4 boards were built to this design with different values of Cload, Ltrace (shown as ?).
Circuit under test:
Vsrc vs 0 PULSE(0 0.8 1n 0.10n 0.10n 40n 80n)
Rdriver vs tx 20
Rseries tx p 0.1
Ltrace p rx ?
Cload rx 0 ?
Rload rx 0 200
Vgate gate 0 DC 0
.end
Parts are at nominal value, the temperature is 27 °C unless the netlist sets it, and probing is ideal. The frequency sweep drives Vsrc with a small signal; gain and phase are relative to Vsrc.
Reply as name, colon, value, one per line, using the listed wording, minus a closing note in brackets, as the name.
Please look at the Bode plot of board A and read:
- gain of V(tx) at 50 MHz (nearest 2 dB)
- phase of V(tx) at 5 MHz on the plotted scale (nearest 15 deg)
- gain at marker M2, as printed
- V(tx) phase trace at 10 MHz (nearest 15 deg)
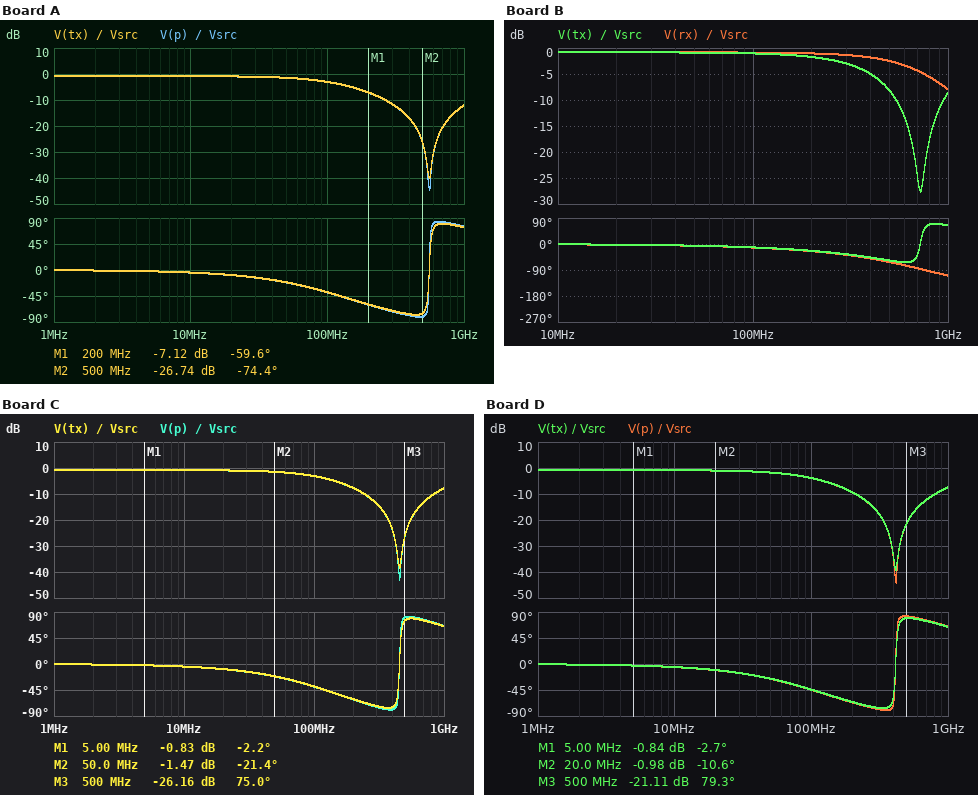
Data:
gain of V(tx) at 50 MHz: -2 dB
phase of V(tx) at 5 MHz on the plotted scale: 0 deg
gain at marker M2, as printed: -26.74 dB
V(tx) phase trace at 10 MHz: 0 deg
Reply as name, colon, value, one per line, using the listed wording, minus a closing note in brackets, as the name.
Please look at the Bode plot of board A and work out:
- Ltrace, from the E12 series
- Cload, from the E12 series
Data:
Ltrace, from the E12 series: 1.2 nH
Cload, from the E12 series: 68 pF
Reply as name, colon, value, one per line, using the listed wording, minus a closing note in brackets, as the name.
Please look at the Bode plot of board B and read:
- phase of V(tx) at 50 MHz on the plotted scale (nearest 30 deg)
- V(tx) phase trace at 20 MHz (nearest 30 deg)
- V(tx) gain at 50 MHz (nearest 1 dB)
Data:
phase of V(tx) at 50 MHz on the plotted scale: 0 deg
V(tx) phase trace at 20 MHz: 0 deg
V(tx) gain at 50 MHz: -1 dB
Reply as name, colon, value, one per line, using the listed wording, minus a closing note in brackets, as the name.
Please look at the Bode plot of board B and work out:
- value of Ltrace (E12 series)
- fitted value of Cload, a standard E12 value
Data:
value of Ltrace: 2.7 nH
fitted value of Cload, a standard E12 value: 18 pF
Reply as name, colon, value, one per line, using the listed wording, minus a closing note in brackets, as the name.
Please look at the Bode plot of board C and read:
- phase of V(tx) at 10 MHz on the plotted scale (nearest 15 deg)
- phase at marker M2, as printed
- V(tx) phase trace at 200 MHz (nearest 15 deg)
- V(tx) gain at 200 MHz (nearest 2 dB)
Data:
phase of V(tx) at 10 MHz on the plotted scale: 0 deg
phase at marker M2, as printed: -21.4 deg
V(tx) phase trace at 200 MHz: -60 deg
V(tx) gain at 200 MHz: -8 dB
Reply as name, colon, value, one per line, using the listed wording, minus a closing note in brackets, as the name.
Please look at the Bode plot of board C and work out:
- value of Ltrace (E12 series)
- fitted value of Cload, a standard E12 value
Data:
value of Ltrace: 1.8 nH
fitted value of Cload, a standard E12 value: 68 pF
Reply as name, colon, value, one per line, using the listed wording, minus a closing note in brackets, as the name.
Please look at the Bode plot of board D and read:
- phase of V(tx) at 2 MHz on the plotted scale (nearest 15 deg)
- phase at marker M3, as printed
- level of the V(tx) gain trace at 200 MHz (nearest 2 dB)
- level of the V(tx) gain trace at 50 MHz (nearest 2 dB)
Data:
phase of V(tx) at 2 MHz on the plotted scale: 0 deg
phase at marker M3, as printed: 79.3 deg
level of the V(tx) gain trace at 200 MHz: -10 dB
level of the V(tx) gain trace at 50 MHz: -2 dB
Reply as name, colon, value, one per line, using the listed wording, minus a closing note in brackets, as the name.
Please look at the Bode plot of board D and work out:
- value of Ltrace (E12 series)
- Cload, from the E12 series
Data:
value of Ltrace: 1.8 nH
Cload, from the E12 series: 82 pF
